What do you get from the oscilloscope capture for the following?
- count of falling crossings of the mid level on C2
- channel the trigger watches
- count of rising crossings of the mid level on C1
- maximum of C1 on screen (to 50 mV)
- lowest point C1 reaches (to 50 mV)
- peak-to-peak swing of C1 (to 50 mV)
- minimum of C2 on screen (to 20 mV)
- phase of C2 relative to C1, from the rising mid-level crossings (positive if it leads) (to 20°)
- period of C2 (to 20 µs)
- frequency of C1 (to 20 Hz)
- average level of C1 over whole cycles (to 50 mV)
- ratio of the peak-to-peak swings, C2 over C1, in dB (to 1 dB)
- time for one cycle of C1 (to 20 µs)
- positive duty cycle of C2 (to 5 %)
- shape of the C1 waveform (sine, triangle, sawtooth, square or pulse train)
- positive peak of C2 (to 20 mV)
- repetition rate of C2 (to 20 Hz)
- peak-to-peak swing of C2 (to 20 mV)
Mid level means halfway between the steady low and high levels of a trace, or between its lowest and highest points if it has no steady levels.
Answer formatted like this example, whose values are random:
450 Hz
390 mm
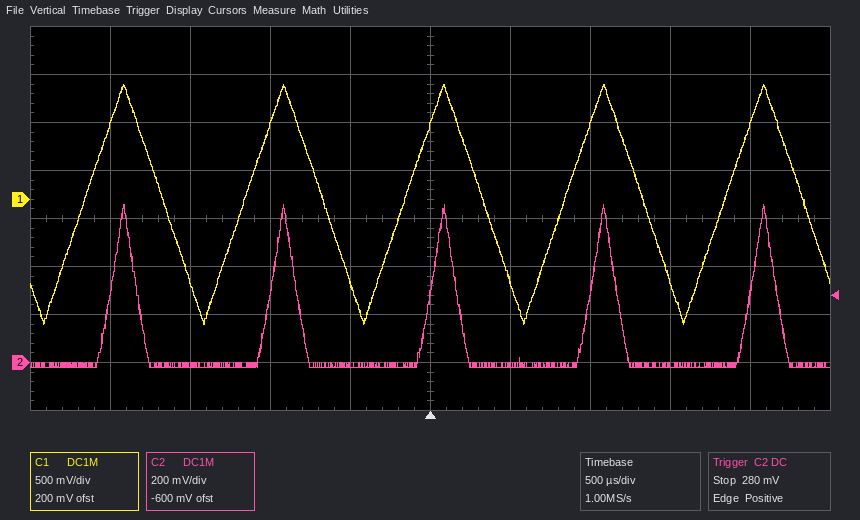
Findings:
5
C2
5
1.20 V
-1.30 V
2.50 V
-20 mV
-60°
1.00 ms
1.00 kHz
-50 mV
-11 dB
1.00 ms
15 %
triangle
660 mV
1.00 kHz
680 mV
